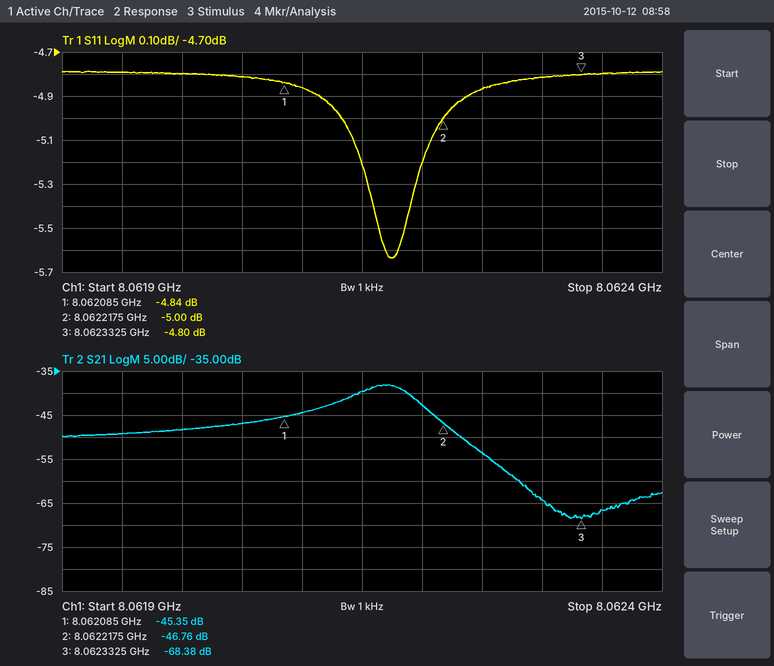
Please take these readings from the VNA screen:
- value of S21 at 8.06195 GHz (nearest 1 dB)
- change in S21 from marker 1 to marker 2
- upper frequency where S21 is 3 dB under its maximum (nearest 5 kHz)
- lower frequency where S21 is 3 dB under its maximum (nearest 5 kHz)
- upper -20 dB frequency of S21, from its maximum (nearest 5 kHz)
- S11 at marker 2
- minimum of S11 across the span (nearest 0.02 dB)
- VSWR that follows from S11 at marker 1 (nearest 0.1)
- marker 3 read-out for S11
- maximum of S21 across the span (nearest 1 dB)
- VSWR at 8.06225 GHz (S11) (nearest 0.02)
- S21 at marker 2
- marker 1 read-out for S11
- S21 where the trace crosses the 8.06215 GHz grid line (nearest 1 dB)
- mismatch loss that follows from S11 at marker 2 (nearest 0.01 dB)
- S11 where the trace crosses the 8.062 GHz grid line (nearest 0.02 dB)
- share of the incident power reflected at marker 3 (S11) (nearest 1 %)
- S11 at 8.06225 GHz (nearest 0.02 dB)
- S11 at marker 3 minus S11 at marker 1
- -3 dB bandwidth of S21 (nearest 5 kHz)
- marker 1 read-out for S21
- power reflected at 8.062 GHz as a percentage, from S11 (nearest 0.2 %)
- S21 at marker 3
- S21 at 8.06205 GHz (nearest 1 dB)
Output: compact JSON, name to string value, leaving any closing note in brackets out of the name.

{"value of S21 at 8.06195 GHz": "-49 dB", "change in S21 from marker 1 to marker 2": "-1.41 dB", "upper frequency where S21 is 3 dB under its maximum": "8.062195 GHz", "lower frequency where S21 is 3 dB under its maximum": "8.062140 GHz", "upper -20 dB frequency of S21, from its maximum": "8.062270 GHz", "S11 at marker 2": "-5.00 dB", "minimum of S11 across the span": "-5.64 dB", "VSWR that follows from S11 at marker 1": "3.7", "marker 3 read-out for S11": "-4.80 dB", "maximum of S21 across the span": "-38 dB", "VSWR at 8.06225 GHz (S11)": "3.66", "S21 at marker 2": "-46.76 dB", "marker 1 read-out for S11": "-4.84 dB", "S21 where the trace crosses the 8.06215 GHz grid line": "-40 dB", "mismatch loss that follows from S11 at marker 2": "1.65 dB", "S11 where the trace crosses the 8.062 GHz grid line": "-4.80 dB", "share of the incident power reflected at marker 3 (S11)": "33 %", "S11 at 8.06225 GHz": "-4.86 dB", "S11 at marker 3 minus S11 at marker 1": "0.04 dB", "-3 dB bandwidth of S21": "55 kHz", "marker 1 read-out for S21": "-45.35 dB", "power reflected at 8.062 GHz as a percentage, from S11": "33.2 %", "S21 at marker 3": "-68.38 dB", "S21 at 8.06205 GHz": "-47 dB"}
